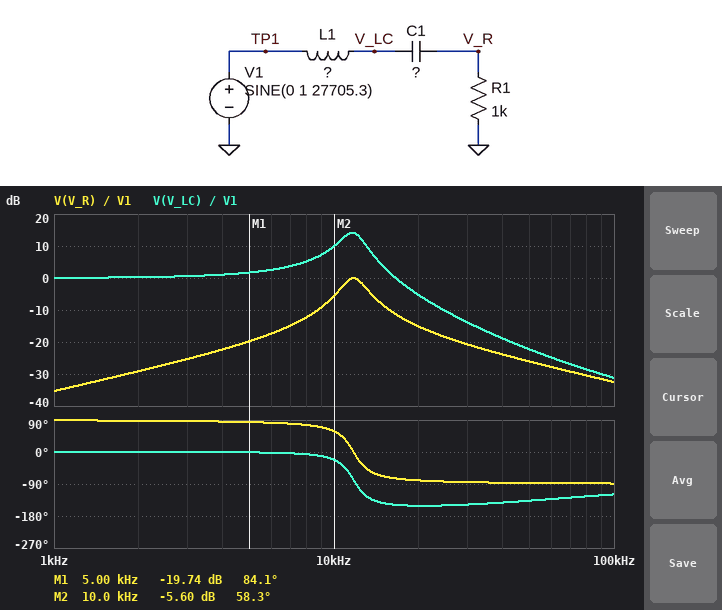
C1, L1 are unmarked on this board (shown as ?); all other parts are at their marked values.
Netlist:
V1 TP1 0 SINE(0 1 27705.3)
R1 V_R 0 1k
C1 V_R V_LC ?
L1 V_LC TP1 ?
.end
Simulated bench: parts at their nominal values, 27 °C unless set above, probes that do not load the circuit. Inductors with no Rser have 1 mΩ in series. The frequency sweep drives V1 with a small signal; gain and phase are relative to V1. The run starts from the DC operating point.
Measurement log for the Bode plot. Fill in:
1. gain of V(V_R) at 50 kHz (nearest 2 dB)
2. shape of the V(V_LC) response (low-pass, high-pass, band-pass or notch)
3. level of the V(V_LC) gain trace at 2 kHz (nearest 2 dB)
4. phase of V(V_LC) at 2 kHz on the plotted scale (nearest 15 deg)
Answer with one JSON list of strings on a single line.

["-26 dB", "low-pass", "0 dB", "0 deg"]
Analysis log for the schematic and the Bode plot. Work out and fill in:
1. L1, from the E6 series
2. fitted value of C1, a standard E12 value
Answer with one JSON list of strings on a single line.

["68 mH", "2.7 nF"]
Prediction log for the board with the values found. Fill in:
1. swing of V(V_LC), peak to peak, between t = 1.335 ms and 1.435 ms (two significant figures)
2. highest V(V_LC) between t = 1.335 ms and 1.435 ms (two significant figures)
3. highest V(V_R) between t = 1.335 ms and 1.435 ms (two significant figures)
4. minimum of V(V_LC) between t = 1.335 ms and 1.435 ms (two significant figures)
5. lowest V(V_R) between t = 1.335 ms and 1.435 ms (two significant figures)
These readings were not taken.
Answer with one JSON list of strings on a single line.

["480 mV", "240 mV", "100 mV", "-240 mV", "-100 mV"]
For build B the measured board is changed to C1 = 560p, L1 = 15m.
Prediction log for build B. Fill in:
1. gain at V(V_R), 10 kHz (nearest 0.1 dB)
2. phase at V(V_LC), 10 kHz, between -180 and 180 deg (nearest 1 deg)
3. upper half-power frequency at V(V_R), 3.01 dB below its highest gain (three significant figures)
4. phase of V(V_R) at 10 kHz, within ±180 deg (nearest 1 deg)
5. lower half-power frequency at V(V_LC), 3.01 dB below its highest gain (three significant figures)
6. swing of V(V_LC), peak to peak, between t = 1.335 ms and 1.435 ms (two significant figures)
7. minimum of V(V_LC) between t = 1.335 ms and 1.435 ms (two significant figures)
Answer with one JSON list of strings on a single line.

["-28.8 dB", "0 deg", "60.5 kHz", "88 deg", "48.8 kHz", "2.7 V", "-1.3 V"]
